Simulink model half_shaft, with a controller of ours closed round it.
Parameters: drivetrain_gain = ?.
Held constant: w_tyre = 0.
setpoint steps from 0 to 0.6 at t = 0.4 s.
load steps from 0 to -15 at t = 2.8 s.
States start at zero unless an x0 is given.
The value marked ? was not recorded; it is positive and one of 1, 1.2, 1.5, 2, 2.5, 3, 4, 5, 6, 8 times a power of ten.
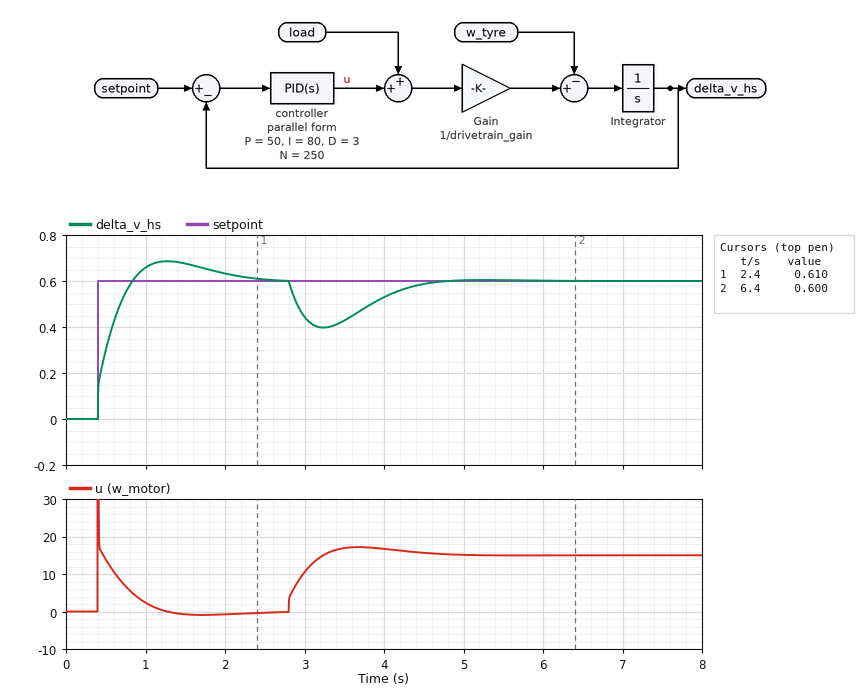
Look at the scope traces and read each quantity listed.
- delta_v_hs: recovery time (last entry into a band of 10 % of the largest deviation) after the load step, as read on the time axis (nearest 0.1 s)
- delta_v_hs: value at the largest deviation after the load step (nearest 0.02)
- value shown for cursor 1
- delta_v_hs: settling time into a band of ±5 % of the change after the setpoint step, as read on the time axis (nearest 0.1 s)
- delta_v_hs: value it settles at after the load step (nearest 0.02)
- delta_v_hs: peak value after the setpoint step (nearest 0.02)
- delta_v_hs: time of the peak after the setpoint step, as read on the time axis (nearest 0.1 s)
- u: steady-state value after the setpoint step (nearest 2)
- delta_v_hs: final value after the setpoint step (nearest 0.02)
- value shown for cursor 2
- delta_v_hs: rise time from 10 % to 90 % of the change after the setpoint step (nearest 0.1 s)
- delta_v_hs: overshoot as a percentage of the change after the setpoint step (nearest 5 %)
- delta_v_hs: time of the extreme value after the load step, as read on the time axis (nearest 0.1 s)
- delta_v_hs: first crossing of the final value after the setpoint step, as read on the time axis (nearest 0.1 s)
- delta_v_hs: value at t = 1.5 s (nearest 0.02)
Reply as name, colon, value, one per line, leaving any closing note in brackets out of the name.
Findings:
delta_v_hs: recovery time (last entry into a band of 10 % of the largest deviation) after the load step, as read on the time axis: 4.4 s
delta_v_hs: value at the largest deviation after the load step: 0.40
value shown for cursor 1: 0.610
delta_v_hs: settling time into a band of ±5 % of the change after the setpoint step, as read on the time axis: 2.0 s
delta_v_hs: value it settles at after the load step: 0.60
delta_v_hs: peak value after the setpoint step: 0.68
delta_v_hs: time of the peak after the setpoint step, as read on the time axis: 1.3 s
u: steady-state value after the setpoint step: 0
delta_v_hs: final value after the setpoint step: 0.60
value shown for cursor 2: 0.600
delta_v_hs: rise time from 10 % to 90 % of the change after the setpoint step: 0.3 s
delta_v_hs: overshoot as a percentage of the change after the setpoint step: 15 %
delta_v_hs: time of the extreme value after the load step, as read on the time axis: 3.2 s
delta_v_hs: first crossing of the final value after the setpoint step, as read on the time axis: 0.8 s
delta_v_hs: value at t = 1.5 s: 0.68
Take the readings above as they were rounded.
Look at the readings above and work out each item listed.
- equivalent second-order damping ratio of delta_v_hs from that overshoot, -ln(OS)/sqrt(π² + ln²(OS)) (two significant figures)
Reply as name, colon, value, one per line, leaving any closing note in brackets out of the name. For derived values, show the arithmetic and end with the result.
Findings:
equivalent second-order damping ratio of delta_v_hs from that overshoot, -ln(OS)/sqrt(π² + ln²(OS)): ln(0.15) = -1.897; 1.897 / sqrt(9.870 + 3.599) = 0.52
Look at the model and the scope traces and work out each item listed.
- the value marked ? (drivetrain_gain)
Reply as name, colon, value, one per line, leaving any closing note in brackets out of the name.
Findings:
the value marked ?: 10
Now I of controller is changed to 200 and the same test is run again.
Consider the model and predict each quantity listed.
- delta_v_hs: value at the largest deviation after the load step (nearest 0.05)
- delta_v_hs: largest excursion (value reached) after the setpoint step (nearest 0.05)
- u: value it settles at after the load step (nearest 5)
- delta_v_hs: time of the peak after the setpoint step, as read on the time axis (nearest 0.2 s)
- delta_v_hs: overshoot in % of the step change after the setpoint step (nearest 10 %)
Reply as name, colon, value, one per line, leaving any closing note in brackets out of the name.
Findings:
delta_v_hs: value at the largest deviation after the load step: 0.45
delta_v_hs: largest excursion (value reached) after the setpoint step: 0.75
u: value it settles at after the load step: 15
delta_v_hs: time of the peak after the setpoint step, as read on the time axis: 1.0 s
delta_v_hs: overshoot in % of the step change after the setpoint step: 20 %
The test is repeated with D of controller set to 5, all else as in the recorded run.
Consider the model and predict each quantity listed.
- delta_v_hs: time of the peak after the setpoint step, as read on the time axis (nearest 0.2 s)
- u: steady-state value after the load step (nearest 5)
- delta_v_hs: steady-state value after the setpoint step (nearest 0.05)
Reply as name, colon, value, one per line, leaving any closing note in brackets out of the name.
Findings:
delta_v_hs: time of the peak after the setpoint step, as read on the time axis: 1.4 s
u: steady-state value after the load step: 15
delta_v_hs: steady-state value after the setpoint step: 0.60
